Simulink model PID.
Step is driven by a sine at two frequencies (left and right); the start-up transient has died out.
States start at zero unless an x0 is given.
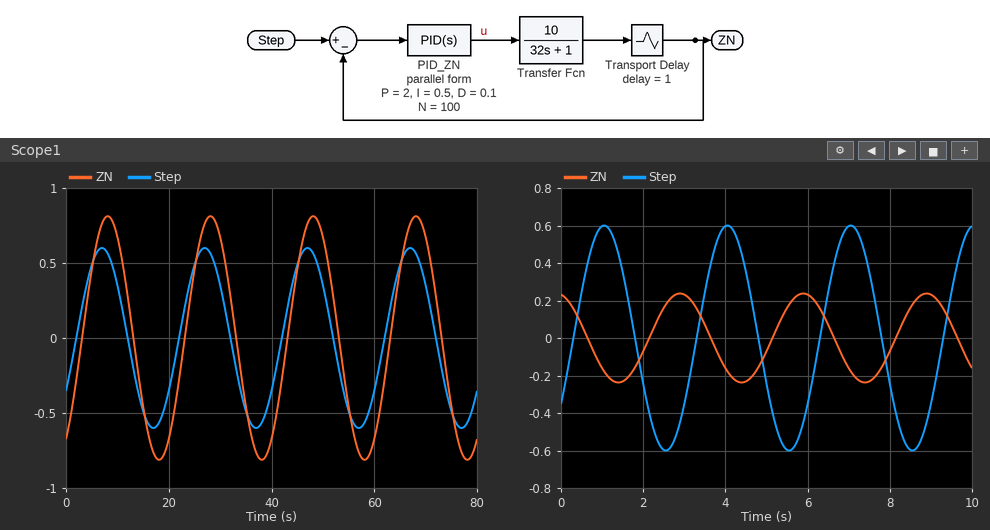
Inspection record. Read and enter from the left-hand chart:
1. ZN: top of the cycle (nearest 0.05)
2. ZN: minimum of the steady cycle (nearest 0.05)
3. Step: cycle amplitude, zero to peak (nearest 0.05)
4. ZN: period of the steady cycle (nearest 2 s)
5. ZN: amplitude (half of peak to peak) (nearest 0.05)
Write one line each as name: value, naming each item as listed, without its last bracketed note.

ZN: top of the cycle: 0.80
ZN: minimum of the steady cycle: -0.80
Step: cycle amplitude, zero to peak: 0.60
ZN: period of the steady cycle: 20 s
ZN: amplitude (half of peak to peak): 0.80
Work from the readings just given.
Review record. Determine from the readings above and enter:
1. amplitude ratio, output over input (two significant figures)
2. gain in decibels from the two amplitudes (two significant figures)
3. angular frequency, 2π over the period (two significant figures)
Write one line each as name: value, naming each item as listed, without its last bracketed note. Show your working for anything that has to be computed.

amplitude ratio, output over input: 0.8 / 0.6 = 1.3
gain in decibels from the two amplitudes: 20 log10(0.8 / 0.6) = 2.5 dB
angular frequency, 2π over the period: 2π / 20 = 0.31 rad/s
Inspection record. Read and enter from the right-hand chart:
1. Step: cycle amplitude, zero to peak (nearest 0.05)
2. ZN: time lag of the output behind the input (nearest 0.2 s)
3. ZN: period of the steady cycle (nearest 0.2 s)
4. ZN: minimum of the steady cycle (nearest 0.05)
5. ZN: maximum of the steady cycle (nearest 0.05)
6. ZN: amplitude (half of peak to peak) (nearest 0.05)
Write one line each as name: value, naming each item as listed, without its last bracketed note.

Step: cycle amplitude, zero to peak: 0.60
ZN: time lag of the output behind the input: 1.8 s
ZN: period of the steady cycle: 3.0 s
ZN: minimum of the steady cycle: -0.25
ZN: maximum of the steady cycle: 0.25
ZN: amplitude (half of peak to peak): 0.25
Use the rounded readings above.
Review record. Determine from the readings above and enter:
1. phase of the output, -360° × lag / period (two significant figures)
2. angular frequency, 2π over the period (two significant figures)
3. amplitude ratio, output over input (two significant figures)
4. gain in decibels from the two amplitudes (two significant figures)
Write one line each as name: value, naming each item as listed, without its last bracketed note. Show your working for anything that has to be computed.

phase of the output, -360° × lag / period: -360 × 1.8 / 3 = -220°
angular frequency, 2π over the period: 2π / 3 = 2.1 rad/s
amplitude ratio, output over input: 0.25 / 0.6 = 0.42
gain in decibels from the two amplitudes: 20 log10(0.25 / 0.6) = -7.6 dB
